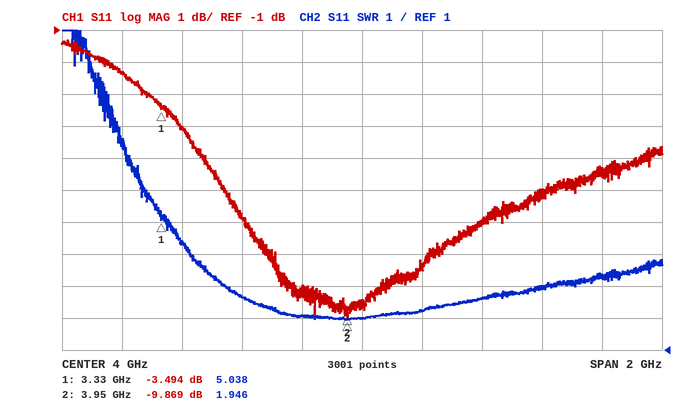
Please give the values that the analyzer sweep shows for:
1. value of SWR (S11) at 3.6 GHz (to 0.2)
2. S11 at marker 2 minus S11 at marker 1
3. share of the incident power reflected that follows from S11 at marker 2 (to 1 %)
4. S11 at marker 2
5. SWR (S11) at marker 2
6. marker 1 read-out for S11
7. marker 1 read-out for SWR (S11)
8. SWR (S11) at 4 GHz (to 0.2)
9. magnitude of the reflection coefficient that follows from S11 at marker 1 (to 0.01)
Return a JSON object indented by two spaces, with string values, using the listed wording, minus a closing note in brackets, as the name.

{
  "value of SWR (S11) at 3.6 GHz": "2.6",
  "S11 at marker 2 minus S11 at marker 1": "-6.375 dB",
  "share of the incident power reflected that follows from S11 at marker 2": "10 %",
  "S11 at marker 2": "-9.869 dB",
  "SWR (S11) at marker 2": "1.946",
  "marker 1 read-out for S11": "-3.494 dB",
  "marker 1 read-out for SWR": "5.038",
  "SWR (S11) at 4 GHz": "2.0",
  "magnitude of the reflection coefficient that follows from S11 at marker 1": "0.67"
}
